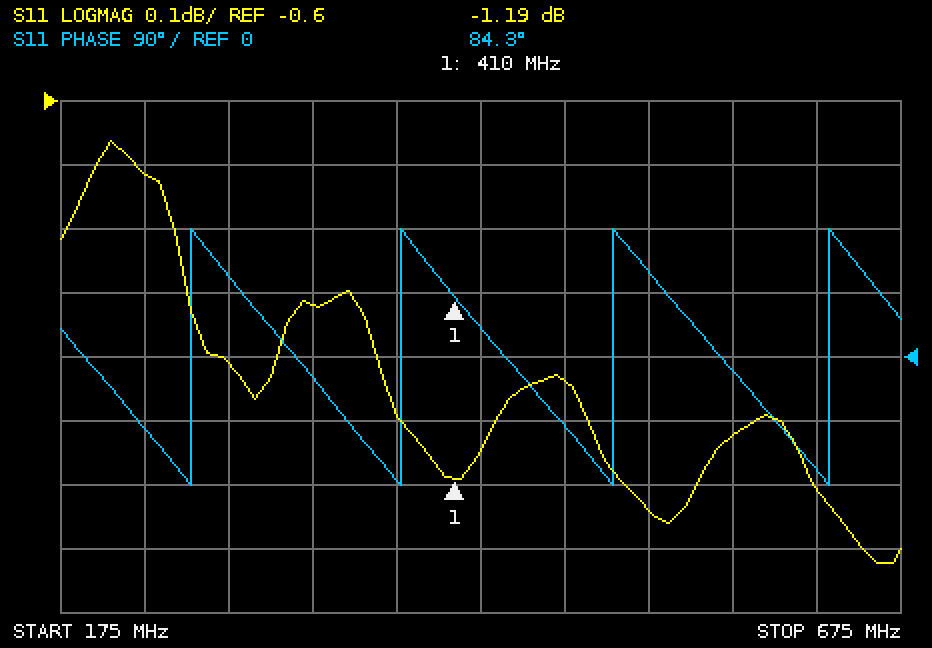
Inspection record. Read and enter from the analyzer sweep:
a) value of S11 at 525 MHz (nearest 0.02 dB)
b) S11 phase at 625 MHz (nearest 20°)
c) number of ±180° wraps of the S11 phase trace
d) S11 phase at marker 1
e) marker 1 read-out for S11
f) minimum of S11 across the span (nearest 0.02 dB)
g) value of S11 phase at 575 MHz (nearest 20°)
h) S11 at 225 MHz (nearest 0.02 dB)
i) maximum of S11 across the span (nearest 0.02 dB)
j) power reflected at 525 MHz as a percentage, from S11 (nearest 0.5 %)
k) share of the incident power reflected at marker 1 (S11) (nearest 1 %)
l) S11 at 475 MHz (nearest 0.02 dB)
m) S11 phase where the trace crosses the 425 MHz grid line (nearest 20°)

-1.24 dB
-160°
4
84.3°
-1.19 dB
-1.32 dB
-20°
-0.72 dB
-0.66 dB
75.0 %
76 %
-1.04 dB
40°
